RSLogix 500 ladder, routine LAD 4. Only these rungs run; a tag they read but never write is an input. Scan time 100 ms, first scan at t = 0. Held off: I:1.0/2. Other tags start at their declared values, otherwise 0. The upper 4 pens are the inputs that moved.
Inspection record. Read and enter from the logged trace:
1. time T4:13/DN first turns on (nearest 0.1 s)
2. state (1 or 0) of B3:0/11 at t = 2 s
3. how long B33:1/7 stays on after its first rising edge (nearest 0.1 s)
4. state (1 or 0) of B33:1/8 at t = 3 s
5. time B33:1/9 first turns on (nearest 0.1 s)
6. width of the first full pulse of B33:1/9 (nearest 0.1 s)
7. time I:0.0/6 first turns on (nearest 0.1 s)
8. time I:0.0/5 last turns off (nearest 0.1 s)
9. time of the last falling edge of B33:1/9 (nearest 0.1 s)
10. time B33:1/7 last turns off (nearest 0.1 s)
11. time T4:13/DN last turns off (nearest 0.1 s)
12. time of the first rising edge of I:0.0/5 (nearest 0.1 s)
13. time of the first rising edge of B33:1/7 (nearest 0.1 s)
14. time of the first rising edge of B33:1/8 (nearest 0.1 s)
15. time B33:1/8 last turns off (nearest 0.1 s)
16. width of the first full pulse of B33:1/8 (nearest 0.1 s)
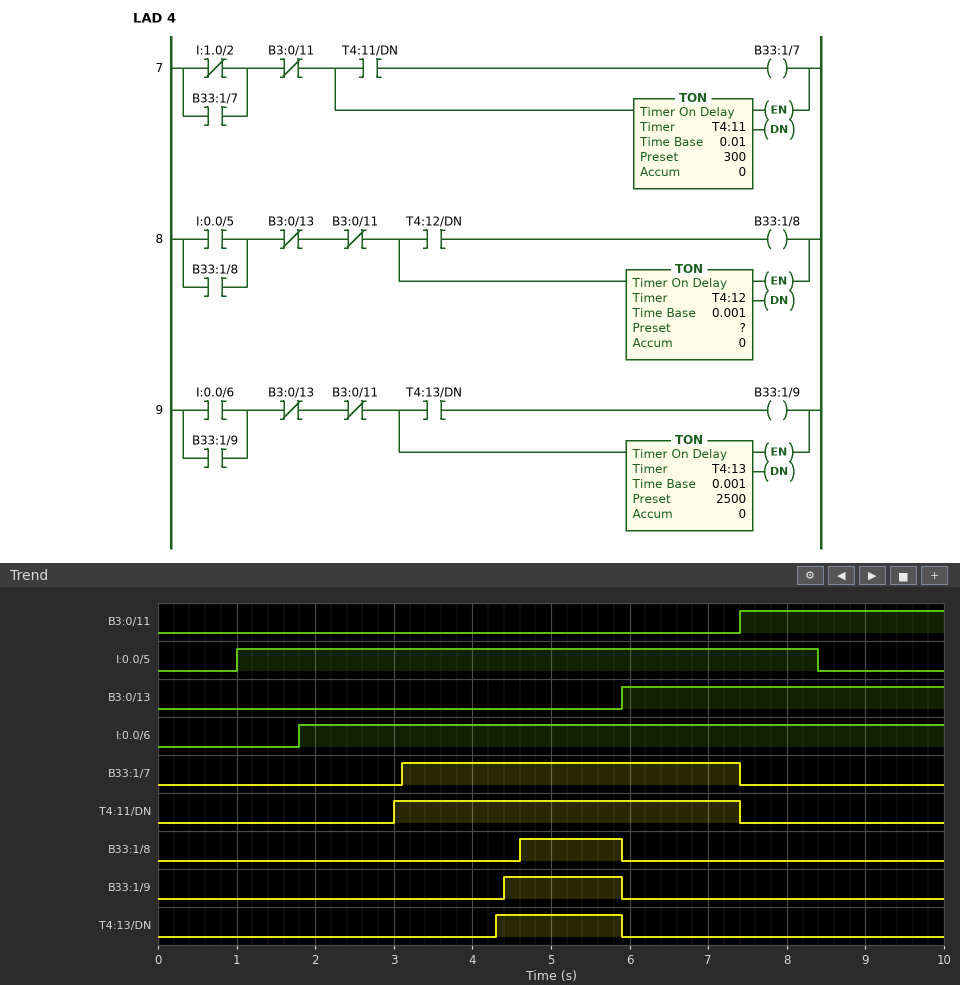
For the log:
4.3 s
0
4.3 s
0
4.4 s
1.5 s
1.8 s
8.4 s
5.9 s
7.4 s
5.9 s
1.0 s
3.1 s
4.6 s
5.9 s
1.3 s
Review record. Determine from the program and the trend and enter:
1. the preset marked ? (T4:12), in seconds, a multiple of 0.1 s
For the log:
3.5 s
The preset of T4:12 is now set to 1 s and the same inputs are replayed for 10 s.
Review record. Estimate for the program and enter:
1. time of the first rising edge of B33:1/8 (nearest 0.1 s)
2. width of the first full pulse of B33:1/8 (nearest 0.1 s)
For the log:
2.1 s
3.8 s
